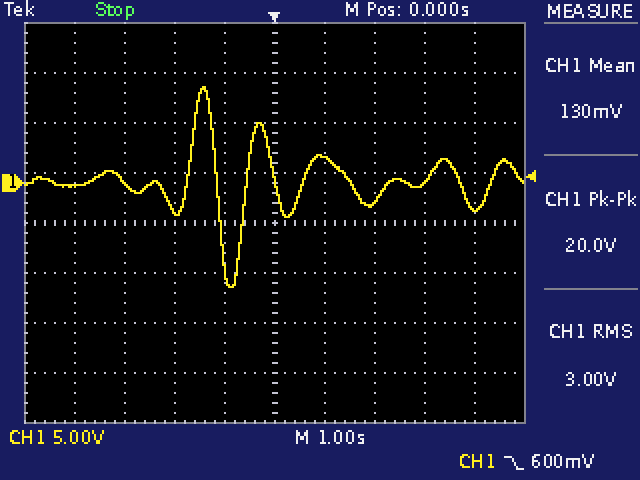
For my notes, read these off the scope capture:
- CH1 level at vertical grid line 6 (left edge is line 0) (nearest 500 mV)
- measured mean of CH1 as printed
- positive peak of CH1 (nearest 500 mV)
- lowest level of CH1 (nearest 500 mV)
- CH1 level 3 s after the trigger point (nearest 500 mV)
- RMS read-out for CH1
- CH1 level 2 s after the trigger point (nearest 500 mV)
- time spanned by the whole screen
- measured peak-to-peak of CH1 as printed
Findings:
2.5 V
130 mV
9.5 V
-10.5 V
0.0 V
3.00 V
-2.0 V
10 s
20.0 V
